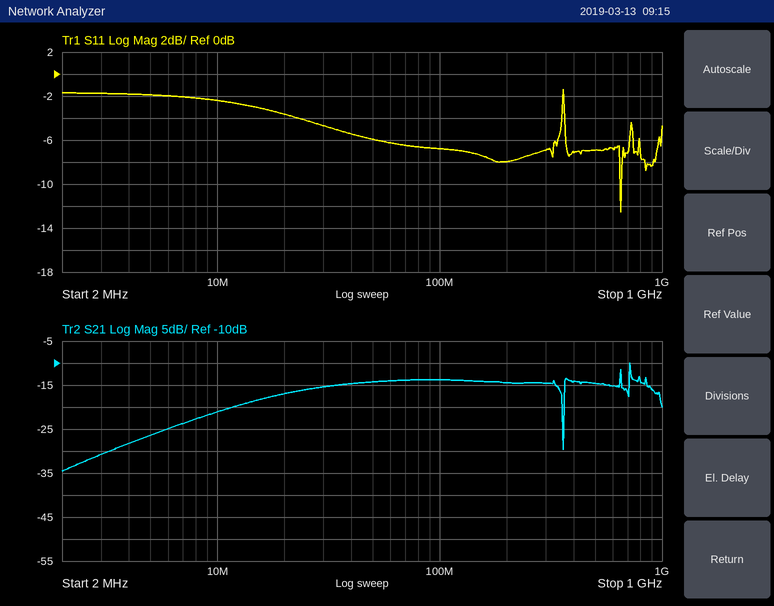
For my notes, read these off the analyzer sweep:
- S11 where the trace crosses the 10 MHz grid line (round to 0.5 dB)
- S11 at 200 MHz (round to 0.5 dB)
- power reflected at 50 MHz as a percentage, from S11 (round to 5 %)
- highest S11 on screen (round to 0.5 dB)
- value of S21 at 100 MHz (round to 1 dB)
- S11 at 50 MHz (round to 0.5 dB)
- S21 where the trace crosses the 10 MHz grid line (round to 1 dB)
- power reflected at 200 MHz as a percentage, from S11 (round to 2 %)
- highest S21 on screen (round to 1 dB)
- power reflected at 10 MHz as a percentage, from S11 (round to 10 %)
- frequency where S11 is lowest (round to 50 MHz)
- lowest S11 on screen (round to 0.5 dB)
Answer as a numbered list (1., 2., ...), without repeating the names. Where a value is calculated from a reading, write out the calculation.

1. -2.5 dB
2. -8.0 dB
3. 10^(-6/10) ≈ 25 %
4. -1.5 dB
5. -14 dB
6. -6.0 dB
7. -21 dB
8. 10^(-8/10) ≈ 16 %
9. -10 dB
10. 10^(-2.5/10) ≈ 56.2 %, so 60 % to the nearest 10 %
11. 650 MHz
12. -12.5 dB
